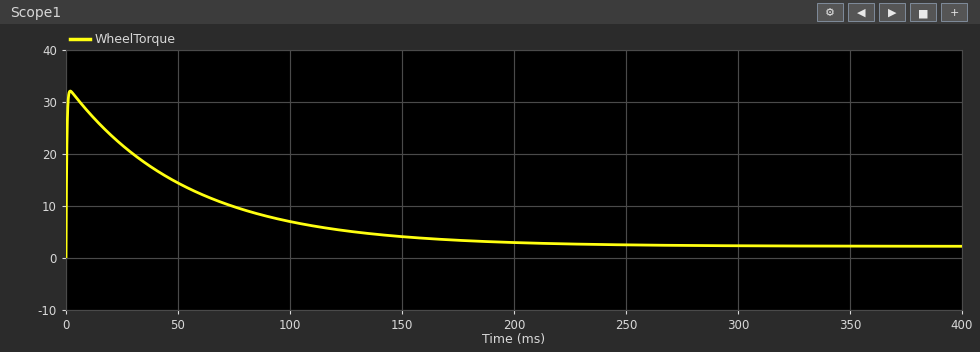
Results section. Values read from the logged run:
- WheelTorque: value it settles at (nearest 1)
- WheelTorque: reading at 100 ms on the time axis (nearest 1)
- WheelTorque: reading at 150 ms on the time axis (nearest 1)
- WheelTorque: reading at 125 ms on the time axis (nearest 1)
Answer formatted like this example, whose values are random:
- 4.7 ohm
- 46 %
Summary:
- 2
- 7
- 4
- 5
